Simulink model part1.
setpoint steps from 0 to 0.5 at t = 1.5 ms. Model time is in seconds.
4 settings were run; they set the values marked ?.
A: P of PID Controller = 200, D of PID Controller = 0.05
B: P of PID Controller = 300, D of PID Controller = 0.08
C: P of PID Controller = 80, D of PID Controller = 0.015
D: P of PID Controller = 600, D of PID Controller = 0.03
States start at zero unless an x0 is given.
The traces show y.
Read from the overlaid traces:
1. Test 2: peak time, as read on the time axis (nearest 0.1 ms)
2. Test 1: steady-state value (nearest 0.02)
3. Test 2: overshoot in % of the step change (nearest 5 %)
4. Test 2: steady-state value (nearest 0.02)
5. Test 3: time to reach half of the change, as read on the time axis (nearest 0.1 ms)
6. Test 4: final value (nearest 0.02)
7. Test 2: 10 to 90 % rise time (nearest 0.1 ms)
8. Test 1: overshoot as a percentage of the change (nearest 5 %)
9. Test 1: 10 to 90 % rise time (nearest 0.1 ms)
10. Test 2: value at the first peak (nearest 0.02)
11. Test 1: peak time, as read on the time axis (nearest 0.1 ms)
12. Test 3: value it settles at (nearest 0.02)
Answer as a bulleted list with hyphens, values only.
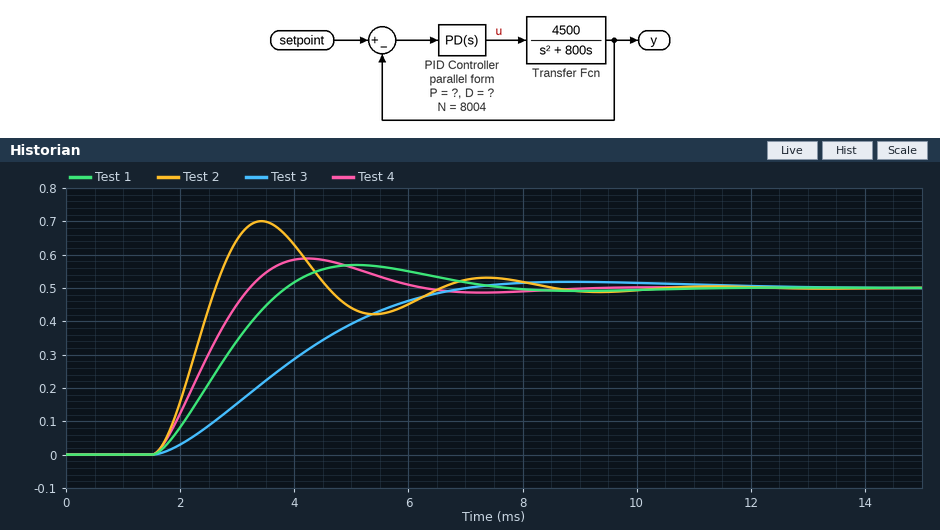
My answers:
- 3.4 ms
- 0.50
- 40 %
- 0.50
- 3.7 ms
- 0.50
- 0.8 ms
- 15 %
- 1.7 ms
- 0.70
- 5.1 ms
- 0.50
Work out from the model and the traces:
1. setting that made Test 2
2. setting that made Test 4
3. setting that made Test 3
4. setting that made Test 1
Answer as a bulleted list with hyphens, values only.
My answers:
- D
- B
- C
- A
